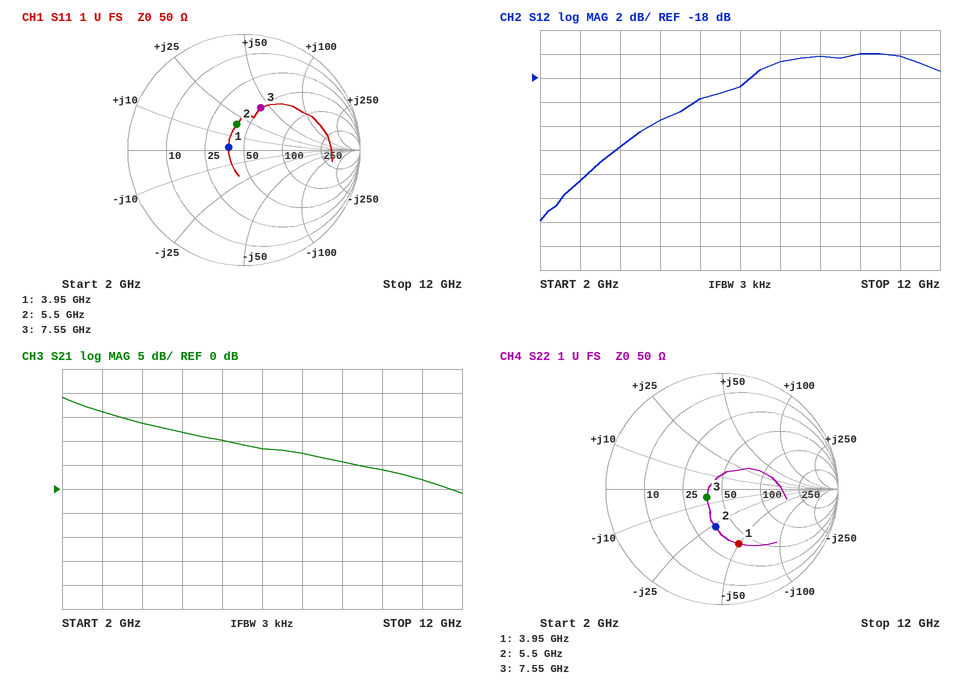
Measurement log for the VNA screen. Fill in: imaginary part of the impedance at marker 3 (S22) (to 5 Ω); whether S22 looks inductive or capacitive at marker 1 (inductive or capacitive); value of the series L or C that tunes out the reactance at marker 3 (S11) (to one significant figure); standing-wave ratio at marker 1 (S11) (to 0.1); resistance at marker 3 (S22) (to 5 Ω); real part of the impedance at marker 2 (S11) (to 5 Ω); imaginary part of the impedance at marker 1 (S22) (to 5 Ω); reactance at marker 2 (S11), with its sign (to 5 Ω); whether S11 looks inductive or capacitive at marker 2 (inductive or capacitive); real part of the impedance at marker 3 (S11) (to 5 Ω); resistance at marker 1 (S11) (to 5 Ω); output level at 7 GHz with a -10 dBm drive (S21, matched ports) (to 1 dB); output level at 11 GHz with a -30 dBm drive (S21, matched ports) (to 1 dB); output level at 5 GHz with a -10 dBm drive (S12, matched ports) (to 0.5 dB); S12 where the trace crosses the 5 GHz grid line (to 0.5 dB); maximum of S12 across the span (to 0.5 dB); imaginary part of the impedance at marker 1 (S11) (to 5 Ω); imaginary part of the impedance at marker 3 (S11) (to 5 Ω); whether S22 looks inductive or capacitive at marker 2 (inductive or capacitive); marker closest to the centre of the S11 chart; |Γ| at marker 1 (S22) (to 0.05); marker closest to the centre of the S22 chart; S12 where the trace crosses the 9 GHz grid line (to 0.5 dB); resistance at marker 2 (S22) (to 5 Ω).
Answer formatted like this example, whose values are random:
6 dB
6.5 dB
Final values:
-5 Ω
capacitive
500 fF
1.3
40 Ω
40 Ω
-50 Ω
+20 Ω
inductive
50 Ω
40 Ω
-2 dBm
-28 dBm
-31.5 dBm
-21.5 dB
-16.0 dB
0 Ω
+40 Ω
capacitive
marker 1
0.50
marker 3
-16.0 dB
35 Ω
